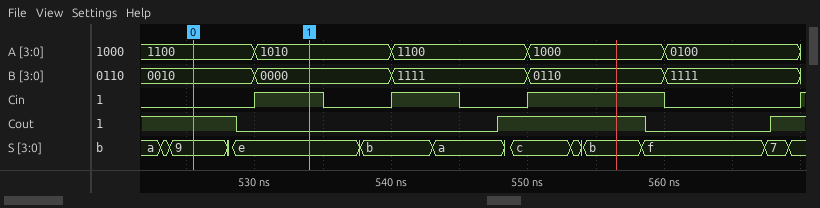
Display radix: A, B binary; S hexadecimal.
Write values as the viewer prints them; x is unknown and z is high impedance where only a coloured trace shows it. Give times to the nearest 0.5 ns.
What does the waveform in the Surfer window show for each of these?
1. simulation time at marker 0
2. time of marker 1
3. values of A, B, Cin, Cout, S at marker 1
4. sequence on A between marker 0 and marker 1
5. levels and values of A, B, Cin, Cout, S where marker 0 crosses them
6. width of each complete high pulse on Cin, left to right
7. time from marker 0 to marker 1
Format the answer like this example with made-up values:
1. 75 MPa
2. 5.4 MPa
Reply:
1. 525.5 ns
2. 534 ns
3. A=1010, B=0000, Cin=1, Cout=0, S=e
4. 1100, 1010
5. A=1100, B=0010, Cin=0, Cout=1, S=9
6. 5 ns, 5 ns, 10 ns
7. 8.5 ns
